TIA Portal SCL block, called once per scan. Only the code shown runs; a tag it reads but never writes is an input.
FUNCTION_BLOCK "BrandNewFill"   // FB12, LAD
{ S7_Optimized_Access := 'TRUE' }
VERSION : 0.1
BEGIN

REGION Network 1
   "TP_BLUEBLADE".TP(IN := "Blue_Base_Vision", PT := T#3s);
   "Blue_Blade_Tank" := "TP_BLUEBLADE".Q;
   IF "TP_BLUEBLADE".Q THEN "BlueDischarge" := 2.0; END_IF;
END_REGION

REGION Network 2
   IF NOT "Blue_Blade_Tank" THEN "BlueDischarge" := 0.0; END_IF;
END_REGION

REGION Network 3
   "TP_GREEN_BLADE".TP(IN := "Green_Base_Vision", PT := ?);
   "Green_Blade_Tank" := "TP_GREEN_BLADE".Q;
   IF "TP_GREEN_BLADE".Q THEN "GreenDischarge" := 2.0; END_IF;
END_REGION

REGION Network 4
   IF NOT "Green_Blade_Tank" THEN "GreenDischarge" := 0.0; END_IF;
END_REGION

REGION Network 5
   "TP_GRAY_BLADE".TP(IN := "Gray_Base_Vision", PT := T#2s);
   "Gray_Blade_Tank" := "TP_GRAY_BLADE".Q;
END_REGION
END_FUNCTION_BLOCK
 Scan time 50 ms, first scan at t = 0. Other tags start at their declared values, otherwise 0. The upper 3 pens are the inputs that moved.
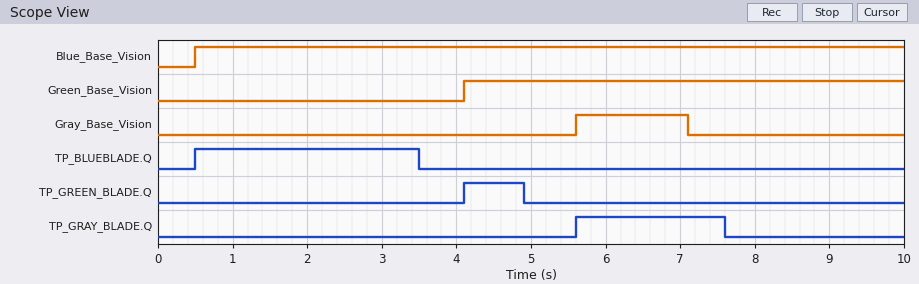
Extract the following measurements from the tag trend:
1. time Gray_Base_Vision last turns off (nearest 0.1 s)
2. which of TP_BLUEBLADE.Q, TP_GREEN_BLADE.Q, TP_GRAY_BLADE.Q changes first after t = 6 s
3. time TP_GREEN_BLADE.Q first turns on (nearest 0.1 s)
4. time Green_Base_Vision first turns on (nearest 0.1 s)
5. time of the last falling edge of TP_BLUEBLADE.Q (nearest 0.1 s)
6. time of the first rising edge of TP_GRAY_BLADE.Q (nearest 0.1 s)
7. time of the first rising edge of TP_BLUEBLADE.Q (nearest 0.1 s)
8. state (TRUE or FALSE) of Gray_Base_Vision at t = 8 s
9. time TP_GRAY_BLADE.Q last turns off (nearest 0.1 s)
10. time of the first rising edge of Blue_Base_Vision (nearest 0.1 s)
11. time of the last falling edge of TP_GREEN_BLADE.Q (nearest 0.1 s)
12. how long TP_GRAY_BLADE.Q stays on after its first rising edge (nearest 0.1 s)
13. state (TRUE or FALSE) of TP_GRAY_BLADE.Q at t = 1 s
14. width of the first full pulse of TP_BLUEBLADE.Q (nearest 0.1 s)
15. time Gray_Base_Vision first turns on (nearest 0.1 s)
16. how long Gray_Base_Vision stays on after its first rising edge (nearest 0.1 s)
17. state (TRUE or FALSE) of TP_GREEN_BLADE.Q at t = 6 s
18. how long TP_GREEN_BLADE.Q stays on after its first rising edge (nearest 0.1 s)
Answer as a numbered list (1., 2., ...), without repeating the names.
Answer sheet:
1. 7.1 s
2. TP_GRAY_BLADE.Q
3. 4.1 s
4. 4.1 s
5. 3.5 s
6. 5.6 s
7. 0.5 s
8. FALSE
9. 7.6 s
10. 0.5 s
11. 4.9 s
12. 2.0 s
13. FALSE
14. 3.0 s
15. 5.6 s
16. 1.5 s
17. FALSE
18. 0.8 s
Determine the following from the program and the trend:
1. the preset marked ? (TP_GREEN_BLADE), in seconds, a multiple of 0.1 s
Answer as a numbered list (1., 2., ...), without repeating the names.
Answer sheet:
1. 0.8 s
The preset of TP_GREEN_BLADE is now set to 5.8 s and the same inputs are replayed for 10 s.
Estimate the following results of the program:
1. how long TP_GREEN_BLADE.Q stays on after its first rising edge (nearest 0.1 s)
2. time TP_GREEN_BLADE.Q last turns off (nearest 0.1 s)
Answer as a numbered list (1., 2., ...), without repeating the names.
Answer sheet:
1. 5.8 s
2. 9.9 s
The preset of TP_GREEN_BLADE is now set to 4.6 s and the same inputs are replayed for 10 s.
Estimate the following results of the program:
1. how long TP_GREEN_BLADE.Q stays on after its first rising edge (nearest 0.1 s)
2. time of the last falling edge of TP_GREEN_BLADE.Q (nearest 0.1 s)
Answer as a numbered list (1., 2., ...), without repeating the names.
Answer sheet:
1. 4.6 s
2. 8.7 s
